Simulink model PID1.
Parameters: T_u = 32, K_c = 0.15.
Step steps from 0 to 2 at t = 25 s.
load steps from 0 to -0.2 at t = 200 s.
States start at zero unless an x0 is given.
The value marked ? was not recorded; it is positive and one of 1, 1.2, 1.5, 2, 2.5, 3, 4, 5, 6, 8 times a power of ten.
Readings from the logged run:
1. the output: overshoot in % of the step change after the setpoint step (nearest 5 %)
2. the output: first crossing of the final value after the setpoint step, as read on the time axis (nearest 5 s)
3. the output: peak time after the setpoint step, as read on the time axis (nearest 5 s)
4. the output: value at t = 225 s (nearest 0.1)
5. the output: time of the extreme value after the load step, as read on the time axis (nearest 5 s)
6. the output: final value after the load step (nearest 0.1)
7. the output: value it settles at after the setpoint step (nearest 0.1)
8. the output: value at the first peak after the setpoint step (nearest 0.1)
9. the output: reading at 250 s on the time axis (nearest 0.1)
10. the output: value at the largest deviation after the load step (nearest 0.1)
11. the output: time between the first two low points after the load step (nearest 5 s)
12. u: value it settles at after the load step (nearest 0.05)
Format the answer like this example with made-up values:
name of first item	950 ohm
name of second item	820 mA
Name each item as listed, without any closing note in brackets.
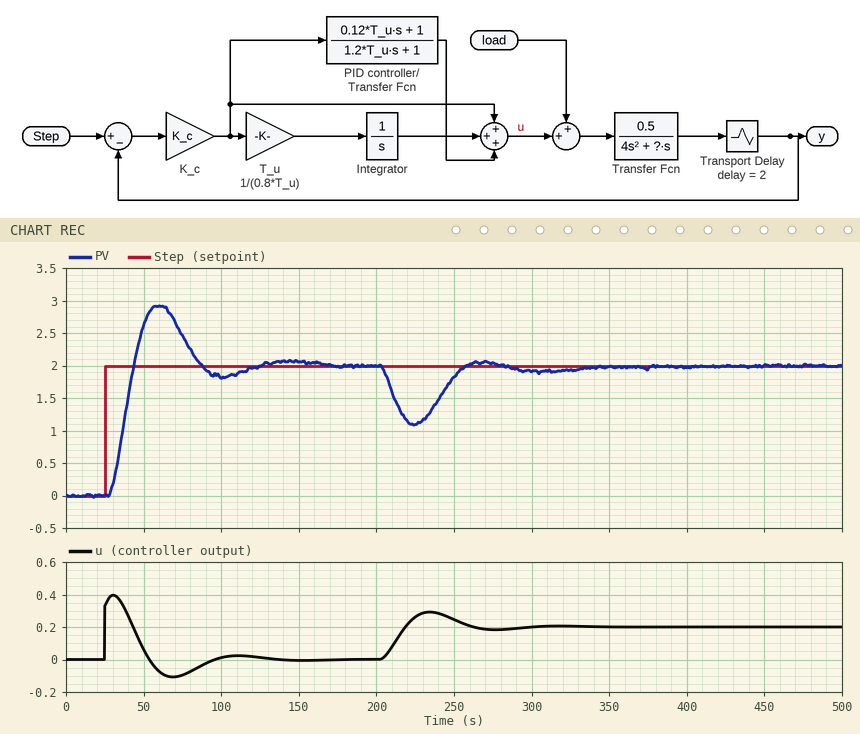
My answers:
the output: overshoot in % of the step change after the setpoint step	45 %
the output: first crossing of the final value after the setpoint step, as read on the time axis	45 s
the output: peak time after the setpoint step, as read on the time axis	60 s
the output: value at t = 225 s	1.1
the output: time of the extreme value after the load step, as read on the time axis	225 s
the output: final value after the load step	2.0
the output: value it settles at after the setpoint step	2.0
the output: value at the first peak after the setpoint step	2.9
the output: reading at 250 s on the time axis	1.8
the output: value at the largest deviation after the load step	1.1
the output: time between the first two low points after the load step	80 s
u: value it settles at after the load step	0.20
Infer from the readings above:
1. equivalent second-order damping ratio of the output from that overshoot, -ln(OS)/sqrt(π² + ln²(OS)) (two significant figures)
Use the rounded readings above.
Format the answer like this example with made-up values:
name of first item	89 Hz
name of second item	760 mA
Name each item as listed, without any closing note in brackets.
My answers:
equivalent second-order damping ratio of the output from that overshoot, -ln(OS)/sqrt(π² + ln²(OS))	0.25
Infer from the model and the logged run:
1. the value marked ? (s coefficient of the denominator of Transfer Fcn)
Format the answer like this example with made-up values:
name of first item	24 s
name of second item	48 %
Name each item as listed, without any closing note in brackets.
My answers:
the value marked ?	1.2
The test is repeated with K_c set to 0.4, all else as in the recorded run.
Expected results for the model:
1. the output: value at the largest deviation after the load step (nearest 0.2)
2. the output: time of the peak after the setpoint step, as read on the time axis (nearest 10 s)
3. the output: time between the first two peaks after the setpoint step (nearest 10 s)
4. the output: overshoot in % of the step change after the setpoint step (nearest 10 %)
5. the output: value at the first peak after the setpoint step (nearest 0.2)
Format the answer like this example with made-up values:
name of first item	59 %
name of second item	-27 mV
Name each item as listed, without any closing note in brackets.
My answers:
the output: value at the largest deviation after the load step	1.4
the output: time of the peak after the setpoint step, as read on the time axis	40 s
the output: time between the first two peaks after the setpoint step	30 s
the output: overshoot in % of the step change after the setpoint step	70 %
the output: value at the first peak after the setpoint step	3.4
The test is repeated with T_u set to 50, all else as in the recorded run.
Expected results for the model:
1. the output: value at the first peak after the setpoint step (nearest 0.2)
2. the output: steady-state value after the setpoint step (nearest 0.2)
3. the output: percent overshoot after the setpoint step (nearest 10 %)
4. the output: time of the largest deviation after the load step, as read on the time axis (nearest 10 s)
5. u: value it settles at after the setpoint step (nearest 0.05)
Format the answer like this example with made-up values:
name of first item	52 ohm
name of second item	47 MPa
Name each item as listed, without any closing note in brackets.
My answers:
the output: value at the first peak after the setpoint step	2.6
the output: steady-state value after the setpoint step	2.0
the output: percent overshoot after the setpoint step	30 %
the output: time of the largest deviation after the load step, as read on the time axis	230 s
u: value it settles at after the setpoint step	0.00
